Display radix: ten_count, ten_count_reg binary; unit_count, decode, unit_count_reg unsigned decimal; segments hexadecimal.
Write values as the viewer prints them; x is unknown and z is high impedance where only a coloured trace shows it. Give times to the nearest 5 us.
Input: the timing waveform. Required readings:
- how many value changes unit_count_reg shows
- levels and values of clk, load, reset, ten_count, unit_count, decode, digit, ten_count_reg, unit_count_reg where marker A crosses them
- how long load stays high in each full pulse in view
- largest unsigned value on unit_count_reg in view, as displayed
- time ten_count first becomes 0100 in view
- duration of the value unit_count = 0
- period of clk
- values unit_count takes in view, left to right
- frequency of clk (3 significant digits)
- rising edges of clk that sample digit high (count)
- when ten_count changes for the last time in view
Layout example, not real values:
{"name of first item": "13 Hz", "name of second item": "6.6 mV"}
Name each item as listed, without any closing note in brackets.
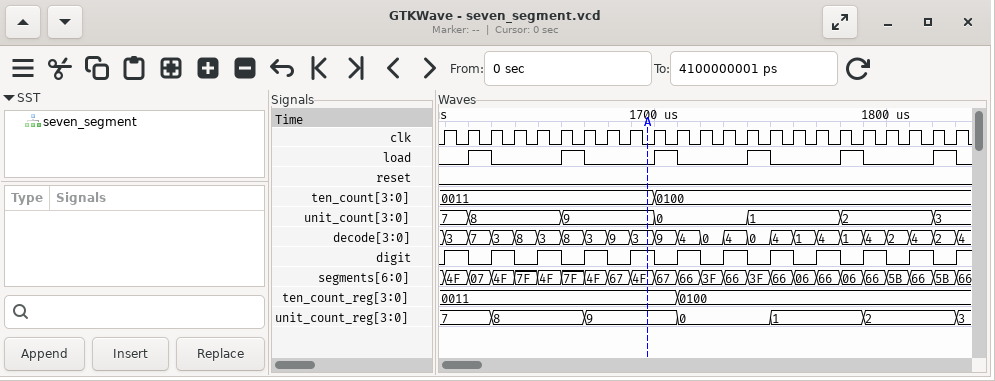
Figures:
{"how many value changes unit_count_reg shows": "6", "levels and values of clk, load, reset, ten_count, unit_count, decode, digit, ten_count_reg, unit_count_reg where marker A crosses them": "clk=0, load=0, reset=0, ten_count=0011, unit_count=9, decode=3, digit=1, ten_count_reg=0011, unit_count_reg=9", "how long load stays high in each full pulse in view": "10 us, 10 us, 10 us, 10 us, 10 us, 10 us", "largest unsigned value on unit_count_reg in view, as displayed": "9", "time ten_count first becomes 0100 in view": "1700 us", "duration of the value unit_count = 0": "40 us", "period of clk": "10 us", "values unit_count takes in view, left to right": "7, 8, 9, 0, 1, 2, 3", "frequency of clk": "100 kHz", "rising edges of clk that sample digit high": "11", "when ten_count changes for the last time in view": "1700 us"}
